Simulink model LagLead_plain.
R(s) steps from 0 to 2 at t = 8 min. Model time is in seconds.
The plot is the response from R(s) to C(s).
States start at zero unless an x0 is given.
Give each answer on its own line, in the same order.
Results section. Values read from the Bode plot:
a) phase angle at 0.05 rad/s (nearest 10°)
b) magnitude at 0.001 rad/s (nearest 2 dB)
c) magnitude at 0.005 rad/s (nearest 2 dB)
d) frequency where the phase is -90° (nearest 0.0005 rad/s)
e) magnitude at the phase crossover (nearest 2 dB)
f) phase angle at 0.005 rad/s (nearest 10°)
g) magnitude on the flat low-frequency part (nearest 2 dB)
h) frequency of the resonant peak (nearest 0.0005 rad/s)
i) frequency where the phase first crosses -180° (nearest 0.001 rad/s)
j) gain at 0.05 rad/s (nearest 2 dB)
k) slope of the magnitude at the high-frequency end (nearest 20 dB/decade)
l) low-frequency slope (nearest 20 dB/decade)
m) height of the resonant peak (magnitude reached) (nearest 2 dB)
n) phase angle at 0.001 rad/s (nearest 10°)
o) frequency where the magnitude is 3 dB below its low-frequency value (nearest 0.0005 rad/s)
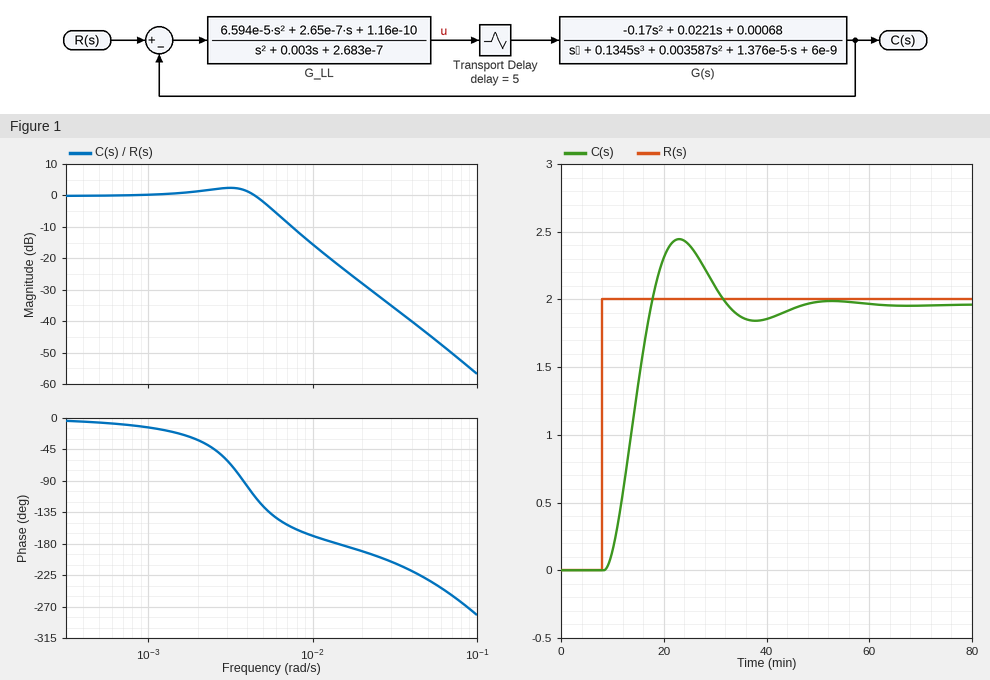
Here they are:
-230°
0 dB
-2 dB
0.0040 rad/s
-22 dB
-130°
0 dB
0.0030 rad/s
0.014 rad/s
-44 dB
-40 dB/decade
0 dB/decade
2 dB
-10°
0.0055 rad/s
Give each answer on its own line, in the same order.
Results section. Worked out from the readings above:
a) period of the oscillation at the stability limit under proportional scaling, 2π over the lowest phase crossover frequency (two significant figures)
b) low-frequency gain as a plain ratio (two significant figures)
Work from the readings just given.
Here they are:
450 s
1.0
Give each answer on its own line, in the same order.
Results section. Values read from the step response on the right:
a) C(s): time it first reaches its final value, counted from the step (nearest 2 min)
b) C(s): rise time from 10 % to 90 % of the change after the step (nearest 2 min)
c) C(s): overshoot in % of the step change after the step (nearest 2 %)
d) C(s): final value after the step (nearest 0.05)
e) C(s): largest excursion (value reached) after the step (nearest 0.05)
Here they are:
10 min
6 min
24 %
1.95
2.45
